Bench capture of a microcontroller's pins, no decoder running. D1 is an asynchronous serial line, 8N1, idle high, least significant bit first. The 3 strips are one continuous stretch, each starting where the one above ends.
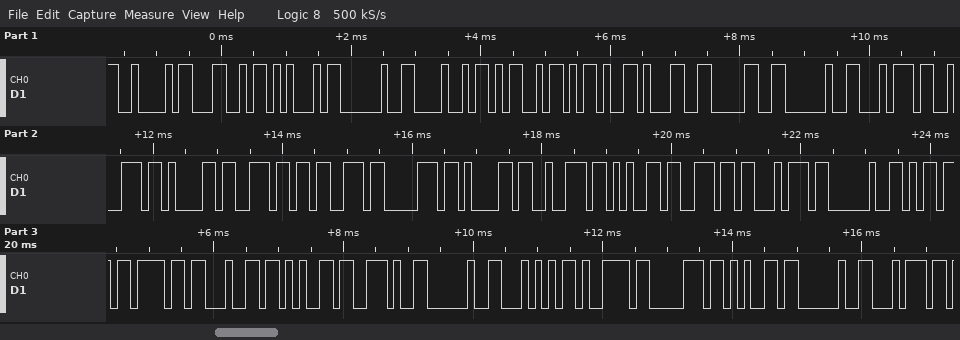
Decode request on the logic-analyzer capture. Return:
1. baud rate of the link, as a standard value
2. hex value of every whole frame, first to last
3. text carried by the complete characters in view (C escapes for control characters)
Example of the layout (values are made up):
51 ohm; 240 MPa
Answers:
9600 baud; 42 4C 45 20 48 4D 2D 31 30 20 74 72 61 6E 73 70 61 72 65 6E 74 20 6D 6F 64 65 2E 20 54 79 70 65 20 74; "BLE HM-10 transparent mode. Type t"
